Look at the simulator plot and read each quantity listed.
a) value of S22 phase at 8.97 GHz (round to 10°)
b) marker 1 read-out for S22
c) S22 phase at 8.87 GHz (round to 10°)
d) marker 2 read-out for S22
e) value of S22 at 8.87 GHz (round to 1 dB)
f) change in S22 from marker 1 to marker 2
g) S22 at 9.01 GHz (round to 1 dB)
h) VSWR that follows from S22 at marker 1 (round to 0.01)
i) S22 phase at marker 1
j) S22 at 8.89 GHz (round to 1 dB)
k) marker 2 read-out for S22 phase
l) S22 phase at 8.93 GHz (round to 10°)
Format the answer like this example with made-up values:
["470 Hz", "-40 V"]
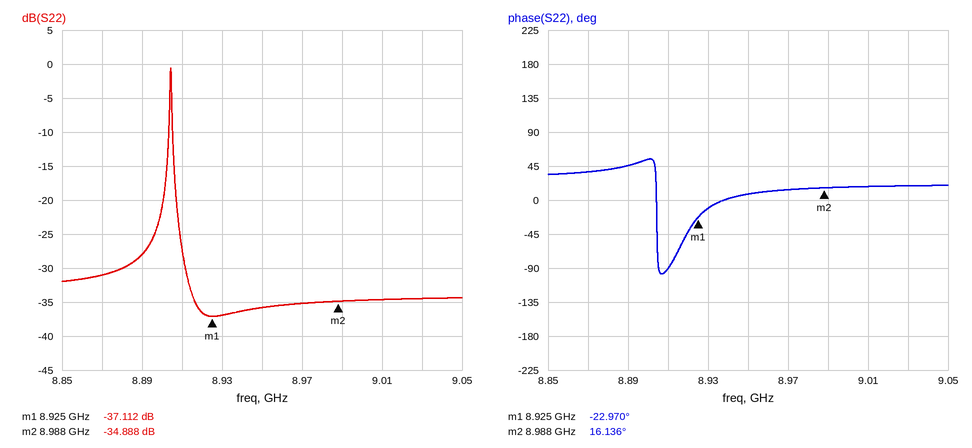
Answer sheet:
["10°", "-37.112 dB", "40°", "-34.888 dB", "-31 dB", "2.224 dB", "-35 dB", "1.03", "-22.970°", "-28 dB", "16.136°", "-10°"]
